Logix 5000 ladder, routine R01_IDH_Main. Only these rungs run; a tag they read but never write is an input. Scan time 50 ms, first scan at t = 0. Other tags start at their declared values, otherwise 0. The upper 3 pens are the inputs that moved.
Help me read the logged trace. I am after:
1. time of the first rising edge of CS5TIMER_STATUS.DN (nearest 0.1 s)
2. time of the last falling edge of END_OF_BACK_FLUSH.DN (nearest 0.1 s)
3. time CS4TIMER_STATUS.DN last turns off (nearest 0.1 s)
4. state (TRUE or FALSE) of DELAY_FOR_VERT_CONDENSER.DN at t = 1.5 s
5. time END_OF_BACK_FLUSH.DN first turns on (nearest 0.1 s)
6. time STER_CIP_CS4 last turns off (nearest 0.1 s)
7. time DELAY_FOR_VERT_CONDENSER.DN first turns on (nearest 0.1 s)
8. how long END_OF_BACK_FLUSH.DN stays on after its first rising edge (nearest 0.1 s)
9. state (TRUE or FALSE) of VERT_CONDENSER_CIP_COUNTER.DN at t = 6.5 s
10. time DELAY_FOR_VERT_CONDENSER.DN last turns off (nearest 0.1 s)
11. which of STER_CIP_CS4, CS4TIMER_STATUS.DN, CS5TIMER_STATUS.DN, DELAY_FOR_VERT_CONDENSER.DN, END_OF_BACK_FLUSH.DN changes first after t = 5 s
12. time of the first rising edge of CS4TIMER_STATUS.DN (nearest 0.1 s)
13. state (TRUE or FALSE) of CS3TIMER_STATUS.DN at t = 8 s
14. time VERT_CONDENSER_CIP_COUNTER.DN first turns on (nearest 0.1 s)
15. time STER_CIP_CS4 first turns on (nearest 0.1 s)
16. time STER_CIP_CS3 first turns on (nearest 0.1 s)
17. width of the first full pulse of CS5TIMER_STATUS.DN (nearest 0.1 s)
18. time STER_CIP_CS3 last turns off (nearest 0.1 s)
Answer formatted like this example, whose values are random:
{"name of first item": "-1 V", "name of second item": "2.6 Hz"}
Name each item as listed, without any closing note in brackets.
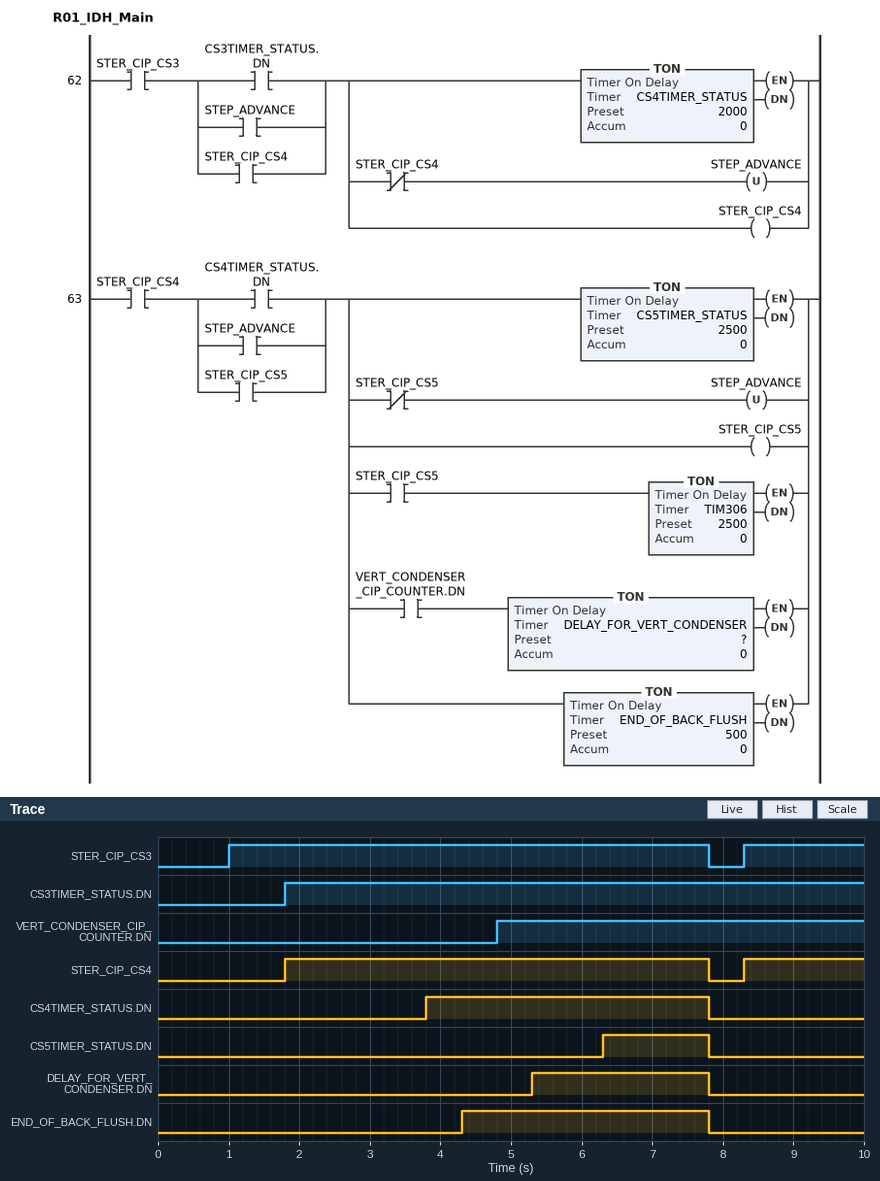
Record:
{"time of the first rising edge of CS5TIMER_STATUS.DN": "6.3 s", "time of the last falling edge of END_OF_BACK_FLUSH.DN": "7.8 s", "time CS4TIMER_STATUS.DN last turns off": "7.8 s", "state (TRUE or FALSE) of DELAY_FOR_VERT_CONDENSER.DN at t = 1.5 s": "FALSE", "time END_OF_BACK_FLUSH.DN first turns on": "4.3 s", "time STER_CIP_CS4 last turns off": "7.8 s", "time DELAY_FOR_VERT_CONDENSER.DN first turns on": "5.3 s", "how long END_OF_BACK_FLUSH.DN stays on after its first rising edge": "3.5 s", "state (TRUE or FALSE) of VERT_CONDENSER_CIP_COUNTER.DN at t = 6.5 s": "TRUE", "time DELAY_FOR_VERT_CONDENSER.DN last turns off": "7.8 s", "which of STER_CIP_CS4, CS4TIMER_STATUS.DN, CS5TIMER_STATUS.DN, DELAY_FOR_VERT_CONDENSER.DN, END_OF_BACK_FLUSH.DN changes first after t = 5 s": "DELAY_FOR_VERT_CONDENSER.DN", "time of the first rising edge of CS4TIMER_STATUS.DN": "3.8 s", "state (TRUE or FALSE) of CS3TIMER_STATUS.DN at t = 8 s": "TRUE", "time VERT_CONDENSER_CIP_COUNTER.DN first turns on": "4.8 s", "time STER_CIP_CS4 first turns on": "1.8 s", "time STER_CIP_CS3 first turns on": "1.0 s", "width of the first full pulse of CS5TIMER_STATUS.DN": "1.5 s", "time STER_CIP_CS3 last turns off": "7.8 s"}
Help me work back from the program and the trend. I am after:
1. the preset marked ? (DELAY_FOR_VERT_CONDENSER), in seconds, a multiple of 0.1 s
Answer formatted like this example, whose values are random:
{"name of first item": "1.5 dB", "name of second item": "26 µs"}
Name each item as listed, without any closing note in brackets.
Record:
{"the preset marked ? (DELAY_FOR_VERT_CONDENSER), in seconds, a multiple of 0.1 s": "0.5 s"}
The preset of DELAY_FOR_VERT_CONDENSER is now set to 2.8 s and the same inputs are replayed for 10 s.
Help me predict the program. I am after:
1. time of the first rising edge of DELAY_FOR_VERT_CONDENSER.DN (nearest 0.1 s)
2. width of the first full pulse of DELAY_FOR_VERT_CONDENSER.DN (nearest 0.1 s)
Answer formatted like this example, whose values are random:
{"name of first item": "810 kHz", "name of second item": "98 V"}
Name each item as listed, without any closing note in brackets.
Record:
{"time of the first rising edge of DELAY_FOR_VERT_CONDENSER.DN": "7.6 s", "width of the first full pulse of DELAY_FOR_VERT_CONDENSER.DN": "0.2 s"}
